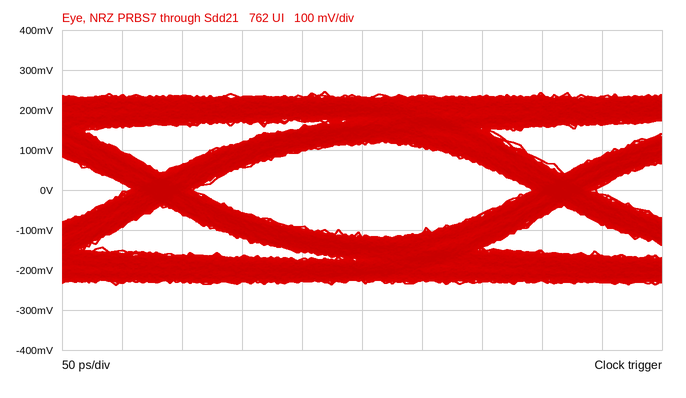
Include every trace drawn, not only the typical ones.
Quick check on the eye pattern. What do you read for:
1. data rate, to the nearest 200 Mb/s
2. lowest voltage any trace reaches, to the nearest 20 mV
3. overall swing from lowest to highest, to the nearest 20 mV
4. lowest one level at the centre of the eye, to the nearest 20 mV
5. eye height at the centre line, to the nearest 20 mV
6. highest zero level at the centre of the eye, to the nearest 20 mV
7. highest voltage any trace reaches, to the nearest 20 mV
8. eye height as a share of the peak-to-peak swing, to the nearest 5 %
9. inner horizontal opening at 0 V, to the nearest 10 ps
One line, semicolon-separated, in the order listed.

3.0 Gb/s; -240 mV; 480 mV; 120 mV; 240 mV; -120 mV; 240 mV; 50 %; 280 ps
